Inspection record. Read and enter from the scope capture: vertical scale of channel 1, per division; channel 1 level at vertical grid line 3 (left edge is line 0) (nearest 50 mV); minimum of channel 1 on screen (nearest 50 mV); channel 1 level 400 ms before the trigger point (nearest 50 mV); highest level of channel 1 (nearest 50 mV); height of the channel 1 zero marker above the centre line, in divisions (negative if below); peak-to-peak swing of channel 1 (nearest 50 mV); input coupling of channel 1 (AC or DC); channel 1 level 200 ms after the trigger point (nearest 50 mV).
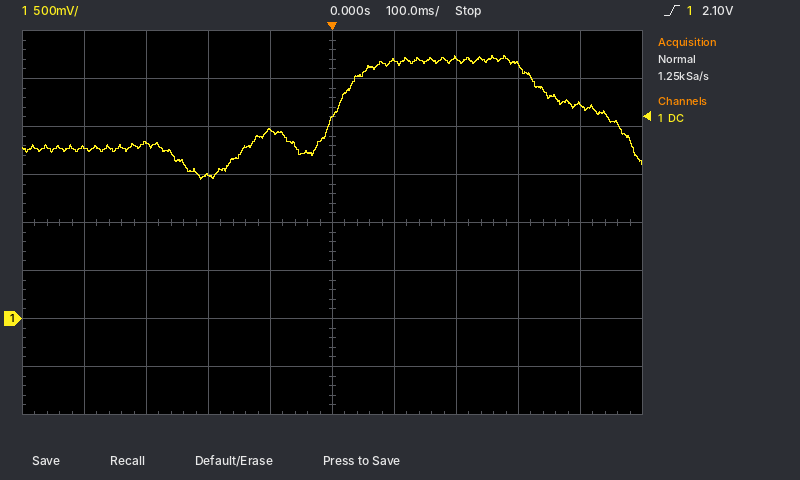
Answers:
500 mV
1.50 V
1.45 V
1.80 V
2.75 V
-2.0 div
1.30 V
DC
2.70 V
